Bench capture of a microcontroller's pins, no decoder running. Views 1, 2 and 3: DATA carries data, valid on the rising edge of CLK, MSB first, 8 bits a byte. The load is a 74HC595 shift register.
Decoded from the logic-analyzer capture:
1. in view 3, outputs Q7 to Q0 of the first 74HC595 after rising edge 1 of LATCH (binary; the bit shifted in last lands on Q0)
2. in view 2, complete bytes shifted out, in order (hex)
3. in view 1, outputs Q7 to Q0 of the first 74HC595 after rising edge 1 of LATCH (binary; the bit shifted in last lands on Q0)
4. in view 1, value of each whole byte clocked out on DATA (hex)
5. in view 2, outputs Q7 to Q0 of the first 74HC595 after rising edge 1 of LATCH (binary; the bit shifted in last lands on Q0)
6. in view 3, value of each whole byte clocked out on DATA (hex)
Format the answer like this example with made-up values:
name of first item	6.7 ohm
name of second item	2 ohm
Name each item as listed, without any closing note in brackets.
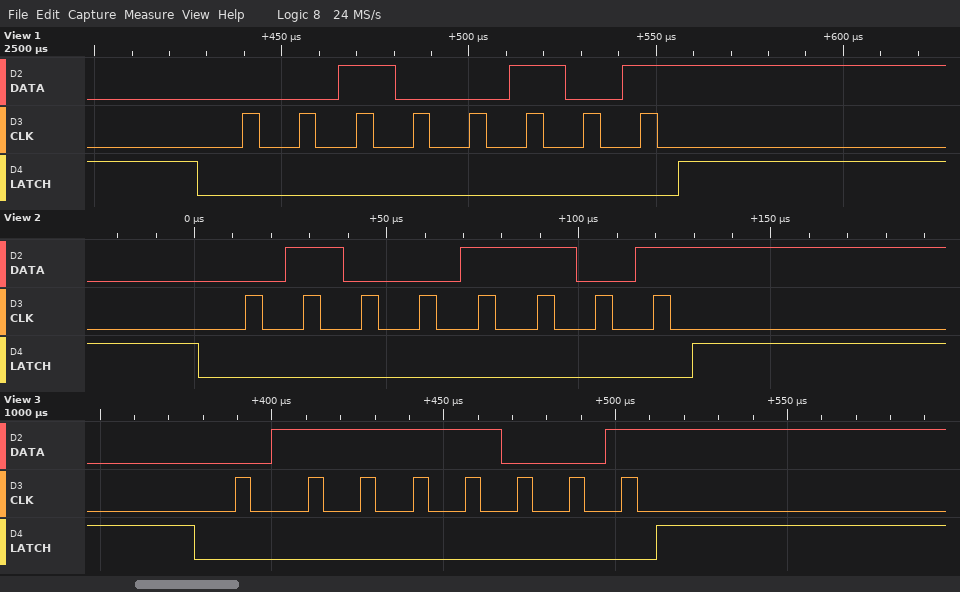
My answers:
in view 3, outputs Q7 to Q0 of the first 74HC595 after rising edge 1 of LATCH	01111001
in view 2, complete bytes shifted out, in order	4D
in view 1, outputs Q7 to Q0 of the first 74HC595 after rising edge 1 of LATCH	00100101
in view 1, value of each whole byte clocked out on DATA	25
in view 2, outputs Q7 to Q0 of the first 74HC595 after rising edge 1 of LATCH	01001101
in view 3, value of each whole byte clocked out on DATA	79
